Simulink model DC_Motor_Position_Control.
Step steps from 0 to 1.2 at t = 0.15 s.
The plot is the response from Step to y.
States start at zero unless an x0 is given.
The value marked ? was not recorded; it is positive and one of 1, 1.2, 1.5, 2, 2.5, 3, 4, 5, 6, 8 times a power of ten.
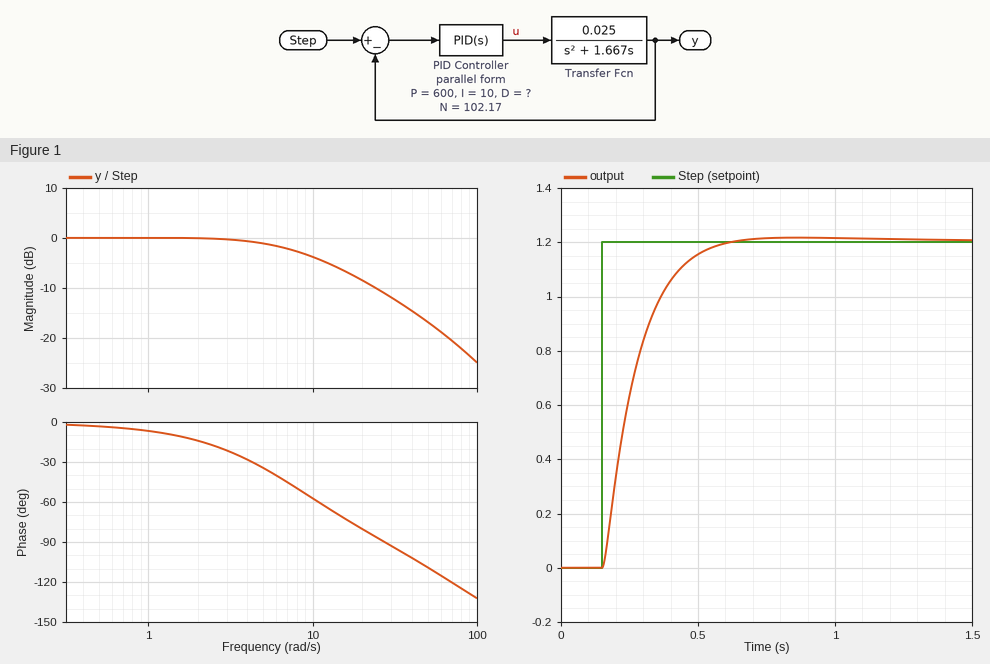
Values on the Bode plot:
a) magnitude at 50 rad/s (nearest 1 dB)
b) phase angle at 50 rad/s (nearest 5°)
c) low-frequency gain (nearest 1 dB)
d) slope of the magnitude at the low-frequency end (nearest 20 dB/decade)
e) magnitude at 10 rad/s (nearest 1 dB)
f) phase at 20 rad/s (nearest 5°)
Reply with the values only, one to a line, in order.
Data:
-17 dB
-110°
0 dB
0 dB/decade
-4 dB
-80°
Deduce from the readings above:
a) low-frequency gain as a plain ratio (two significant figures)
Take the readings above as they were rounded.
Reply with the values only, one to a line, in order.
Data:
1.0
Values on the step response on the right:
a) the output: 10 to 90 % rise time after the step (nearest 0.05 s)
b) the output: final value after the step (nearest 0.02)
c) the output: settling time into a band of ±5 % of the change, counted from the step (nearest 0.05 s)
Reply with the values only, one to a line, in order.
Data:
0.25 s
1.20
0.35 s
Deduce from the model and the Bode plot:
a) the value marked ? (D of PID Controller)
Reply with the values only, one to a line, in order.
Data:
300
